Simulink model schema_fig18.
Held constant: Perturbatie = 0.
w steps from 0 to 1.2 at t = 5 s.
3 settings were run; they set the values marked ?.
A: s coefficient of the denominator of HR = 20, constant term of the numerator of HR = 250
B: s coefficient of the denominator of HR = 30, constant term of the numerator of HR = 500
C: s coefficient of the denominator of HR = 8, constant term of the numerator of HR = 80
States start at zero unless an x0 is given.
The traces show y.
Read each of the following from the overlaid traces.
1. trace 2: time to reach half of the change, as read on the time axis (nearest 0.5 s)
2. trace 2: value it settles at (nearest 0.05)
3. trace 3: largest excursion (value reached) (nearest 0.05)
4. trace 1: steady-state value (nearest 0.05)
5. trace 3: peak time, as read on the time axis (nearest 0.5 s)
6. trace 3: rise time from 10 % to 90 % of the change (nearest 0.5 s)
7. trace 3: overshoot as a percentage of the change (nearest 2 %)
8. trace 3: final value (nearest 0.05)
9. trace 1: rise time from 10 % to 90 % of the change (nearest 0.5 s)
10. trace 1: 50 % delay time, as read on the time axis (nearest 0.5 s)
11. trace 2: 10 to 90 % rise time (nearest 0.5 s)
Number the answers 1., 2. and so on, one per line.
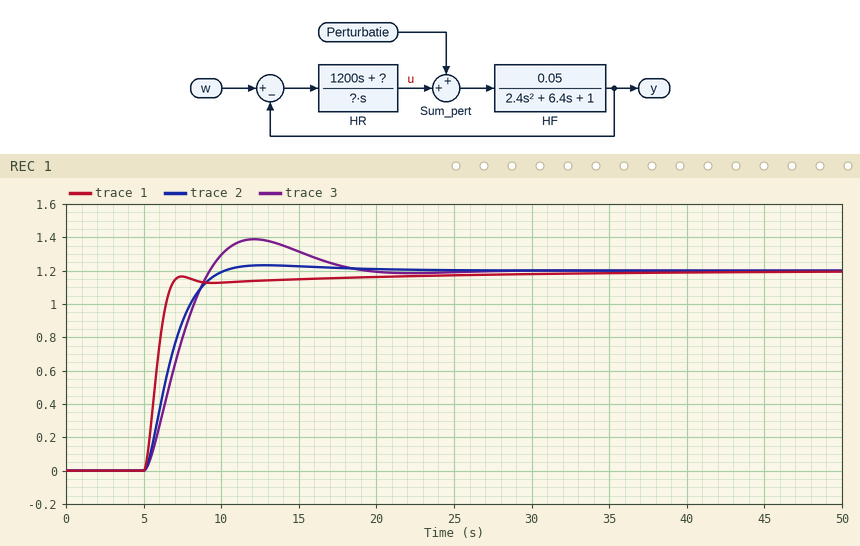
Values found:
1. 6.5 s
2. 1.20
3. 1.40
4. 1.20
5. 12.0 s
6. 3.0 s
7. 16 %
8. 1.20
9. 1.5 s
10. 6.0 s
11. 3.0 s
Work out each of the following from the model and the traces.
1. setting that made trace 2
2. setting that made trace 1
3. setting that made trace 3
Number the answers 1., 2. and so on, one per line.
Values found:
1. A
2. C
3. B
